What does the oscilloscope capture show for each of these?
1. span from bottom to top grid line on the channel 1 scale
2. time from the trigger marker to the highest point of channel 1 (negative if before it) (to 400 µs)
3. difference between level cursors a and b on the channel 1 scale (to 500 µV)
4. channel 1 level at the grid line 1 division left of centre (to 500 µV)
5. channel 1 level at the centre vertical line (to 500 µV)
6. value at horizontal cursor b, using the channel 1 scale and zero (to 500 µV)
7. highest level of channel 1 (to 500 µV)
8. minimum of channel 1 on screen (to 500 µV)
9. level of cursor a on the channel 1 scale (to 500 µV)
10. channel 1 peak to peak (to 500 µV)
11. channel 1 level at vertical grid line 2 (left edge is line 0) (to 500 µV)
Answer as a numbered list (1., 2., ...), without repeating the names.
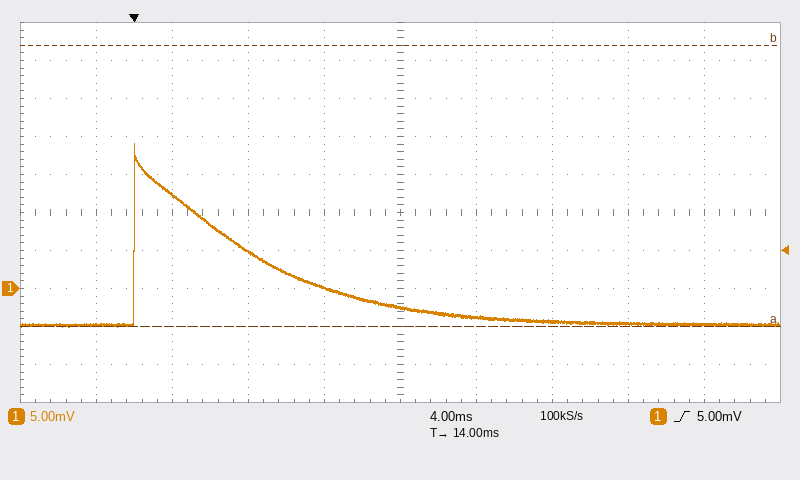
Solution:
1. 50 mV
2. 0.0 ms
3. 37.0 mV
4. 0.0 mV
5. -2.5 mV
6. 32.0 mV
7. 19.0 mV
8. -5.0 mV
9. -5.0 mV
10. 24.0 mV
11. 12.5 mV
